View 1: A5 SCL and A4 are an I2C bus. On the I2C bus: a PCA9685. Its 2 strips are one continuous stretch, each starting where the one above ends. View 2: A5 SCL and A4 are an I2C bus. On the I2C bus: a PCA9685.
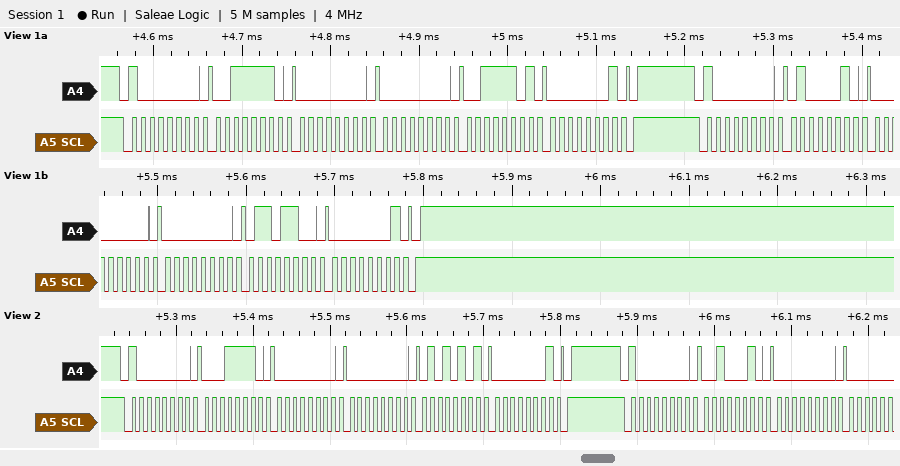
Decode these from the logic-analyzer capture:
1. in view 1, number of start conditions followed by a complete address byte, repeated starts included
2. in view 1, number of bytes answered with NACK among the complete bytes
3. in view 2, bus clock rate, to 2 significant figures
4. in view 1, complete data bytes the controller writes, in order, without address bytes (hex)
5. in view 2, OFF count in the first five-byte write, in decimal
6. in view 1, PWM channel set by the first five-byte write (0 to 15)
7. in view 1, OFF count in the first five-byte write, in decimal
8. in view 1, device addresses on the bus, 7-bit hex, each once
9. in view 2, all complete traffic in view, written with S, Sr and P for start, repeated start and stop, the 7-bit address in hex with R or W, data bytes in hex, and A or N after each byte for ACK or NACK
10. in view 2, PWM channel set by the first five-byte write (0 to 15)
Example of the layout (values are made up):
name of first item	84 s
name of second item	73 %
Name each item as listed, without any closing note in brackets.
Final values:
in view 1, number of start conditions followed by a complete address byte, repeated starts included	2
in view 1, number of bytes answered with NACK among the complete bytes	0
in view 2, bus clock rate, to 2 significant figures	100 kHz
in view 1, complete data bytes the controller writes, in order, without address bytes	3E 00 00 3D 01 42 00 00 6C 01
in view 2, OFF count in the first five-byte write, in decimal	341
in view 1, PWM channel set by the first five-byte write	14
in view 1, OFF count in the first five-byte write, in decimal	317
in view 1, device addresses on the bus, 7-bit hex, each once	0x40
in view 2, all complete traffic in view, written with S, Sr and P for start, repeated start and stop, the 7-bit address in hex with R or W, data bytes in hex, and A or N after each byte for ACK or NACK	S 40W A 1E A 00 A 00 A 55 A 01 A P S 40W A 22 A 00 A
in view 2, PWM channel set by the first five-byte write	6
